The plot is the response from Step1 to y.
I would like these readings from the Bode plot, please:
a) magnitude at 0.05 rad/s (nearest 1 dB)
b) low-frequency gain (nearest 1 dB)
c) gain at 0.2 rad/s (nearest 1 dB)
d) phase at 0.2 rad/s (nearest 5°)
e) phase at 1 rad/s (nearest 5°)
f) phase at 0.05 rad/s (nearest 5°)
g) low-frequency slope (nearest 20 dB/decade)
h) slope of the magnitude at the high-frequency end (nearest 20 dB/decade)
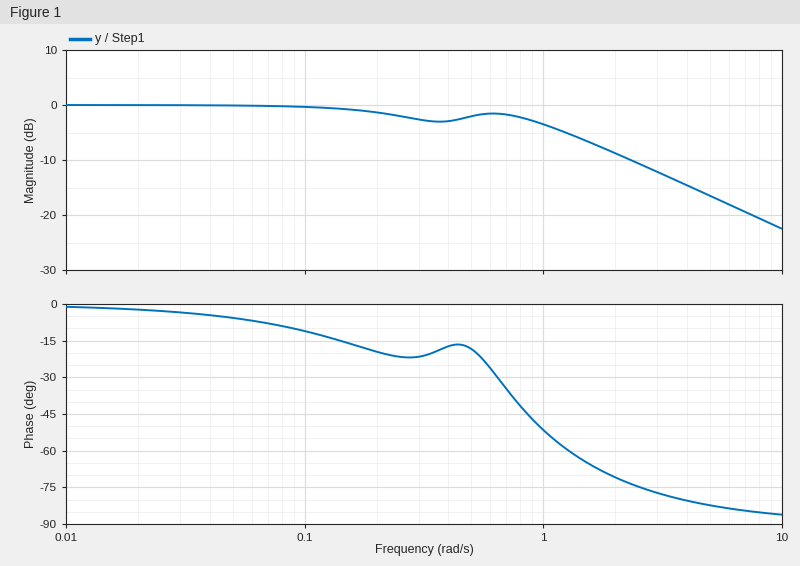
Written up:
0 dB
0 dB
-1 dB
-20°
-50°
-5°
0 dB/decade
-20 dB/decade
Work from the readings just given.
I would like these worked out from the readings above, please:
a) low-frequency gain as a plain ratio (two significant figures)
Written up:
1.0
